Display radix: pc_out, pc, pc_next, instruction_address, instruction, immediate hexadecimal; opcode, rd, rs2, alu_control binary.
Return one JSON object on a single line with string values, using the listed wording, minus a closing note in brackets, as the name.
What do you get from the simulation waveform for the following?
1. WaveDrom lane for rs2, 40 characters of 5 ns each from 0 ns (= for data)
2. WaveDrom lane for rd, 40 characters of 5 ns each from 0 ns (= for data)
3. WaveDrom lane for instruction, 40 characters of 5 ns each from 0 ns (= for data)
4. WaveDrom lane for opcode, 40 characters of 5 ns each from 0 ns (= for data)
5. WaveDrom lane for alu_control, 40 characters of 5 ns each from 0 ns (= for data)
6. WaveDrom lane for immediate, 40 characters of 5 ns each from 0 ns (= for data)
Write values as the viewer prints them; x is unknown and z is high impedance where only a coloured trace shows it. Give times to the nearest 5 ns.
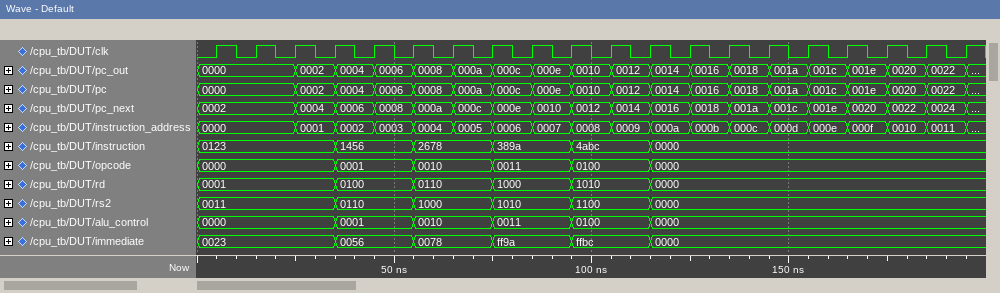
{"WaveDrom lane for rs2, 40 characters of 5 ns each from 0 ns": "{name: 'rs2', wave: '=......=...=...=...=...=................', data: '0011 0110 1000 1010 1100 0000'}", "WaveDrom lane for rd, 40 characters of 5 ns each from 0 ns": "{name: 'rd', wave: '=......=...=...=...=...=................', data: '0001 0100 0110 1000 1010 0000'}", "WaveDrom lane for instruction, 40 characters of 5 ns each from 0 ns": "{name: 'instruction', wave: '=......=...=...=...=...=................', data: '0123 1456 2678 389a 4abc 0000'}", "WaveDrom lane for opcode, 40 characters of 5 ns each from 0 ns": "{name: 'opcode', wave: '=......=...=...=...=...=................', data: '0000 0001 0010 0011 0100 0000'}", "WaveDrom lane for alu_control, 40 characters of 5 ns each from 0 ns": "{name: 'alu_control', wave: '=......=...=...=...=...=................', data: '0000 0001 0010 0011 0100 0000'}", "WaveDrom lane for immediate, 40 characters of 5 ns each from 0 ns": "{name: 'immediate', wave: '=......=...=...=...=...=................', data: '0023 0056 0078 ff9a ffbc 0000'}"}
